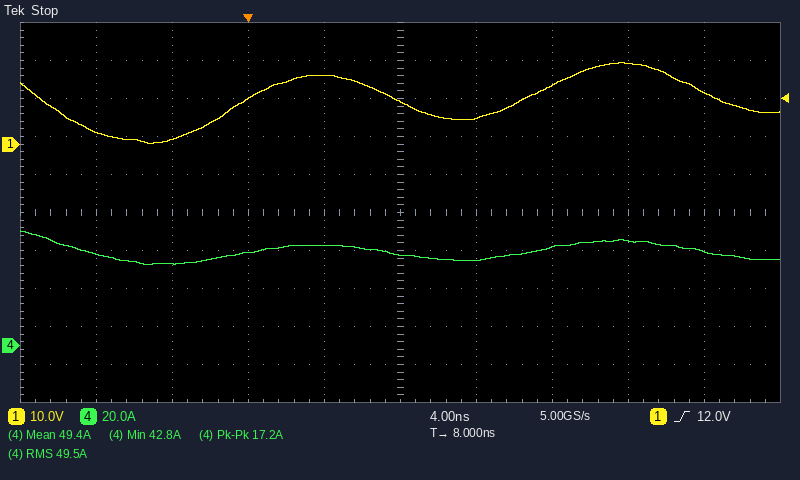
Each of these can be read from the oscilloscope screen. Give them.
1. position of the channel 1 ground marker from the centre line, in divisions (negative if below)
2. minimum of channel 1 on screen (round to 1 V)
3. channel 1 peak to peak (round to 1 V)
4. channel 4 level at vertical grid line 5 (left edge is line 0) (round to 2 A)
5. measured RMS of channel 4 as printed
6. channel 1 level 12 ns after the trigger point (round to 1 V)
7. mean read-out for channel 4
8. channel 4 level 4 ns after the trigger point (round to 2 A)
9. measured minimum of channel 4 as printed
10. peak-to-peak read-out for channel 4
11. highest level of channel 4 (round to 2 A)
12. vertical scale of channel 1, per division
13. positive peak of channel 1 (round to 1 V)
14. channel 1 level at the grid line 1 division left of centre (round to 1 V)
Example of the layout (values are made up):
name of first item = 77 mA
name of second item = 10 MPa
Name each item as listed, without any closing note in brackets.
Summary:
position of the channel 1 ground marker from the centre line, in divisions = +1.8 div
minimum of channel 1 on screen = 0 V
channel 1 peak to peak = 21 V
channel 4 level at vertical grid line 5 (left edge is line 0) = 48 A
measured RMS of channel 4 as printed = 49.5 A
channel 1 level 12 ns after the trigger point = 7 V
mean read-out for channel 4 = 49.4 A
channel 4 level 4 ns after the trigger point = 52 A
measured minimum of channel 4 as printed = 42.8 A
peak-to-peak read-out for channel 4 = 17.2 A
highest level of channel 4 = 60 A
vertical scale of channel 1, per division = 10 V
positive peak of channel 1 = 21 V
channel 1 level at the grid line 1 division left of centre = 18 V
